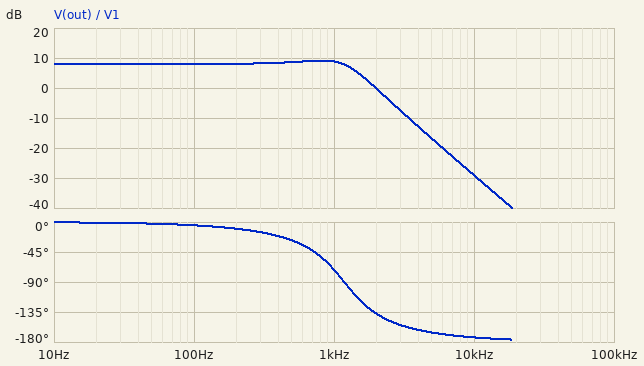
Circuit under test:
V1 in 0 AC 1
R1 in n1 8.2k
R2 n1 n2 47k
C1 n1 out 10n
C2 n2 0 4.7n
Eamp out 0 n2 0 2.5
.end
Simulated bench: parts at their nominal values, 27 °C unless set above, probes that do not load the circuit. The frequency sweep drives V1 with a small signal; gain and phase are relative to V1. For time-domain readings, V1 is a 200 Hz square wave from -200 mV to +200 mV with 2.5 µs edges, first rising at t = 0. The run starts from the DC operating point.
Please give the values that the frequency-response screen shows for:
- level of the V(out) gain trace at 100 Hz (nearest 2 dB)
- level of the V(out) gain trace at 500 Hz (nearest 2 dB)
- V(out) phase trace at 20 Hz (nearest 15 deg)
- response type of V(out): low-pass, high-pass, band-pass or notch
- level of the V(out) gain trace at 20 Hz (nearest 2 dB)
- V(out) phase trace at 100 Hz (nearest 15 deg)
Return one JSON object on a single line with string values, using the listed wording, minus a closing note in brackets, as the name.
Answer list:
{"level of the V(out) gain trace at 100 Hz": "8 dB", "level of the V(out) gain trace at 500 Hz": "8 dB", "V(out) phase trace at 20 Hz": "0 deg", "response type of V(out): low-pass, high-pass, band-pass or notch": "low-pass", "level of the V(out) gain trace at 20 Hz": "8 dB", "V(out) phase trace at 100 Hz": "0 deg"}
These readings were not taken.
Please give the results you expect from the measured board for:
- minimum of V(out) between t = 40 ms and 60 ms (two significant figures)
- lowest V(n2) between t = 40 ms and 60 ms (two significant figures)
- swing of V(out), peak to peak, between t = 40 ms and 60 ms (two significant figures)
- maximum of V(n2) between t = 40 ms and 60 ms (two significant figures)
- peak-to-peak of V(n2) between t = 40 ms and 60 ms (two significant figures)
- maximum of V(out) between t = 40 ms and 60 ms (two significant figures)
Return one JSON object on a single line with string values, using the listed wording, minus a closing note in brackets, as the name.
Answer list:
{"minimum of V(out) between t = 40 ms and 60 ms": "-660 mV", "lowest V(n2) between t = 40 ms and 60 ms": "-260 mV", "swing of V(out), peak to peak, between t = 40 ms and 60 ms": "1.3 V", "maximum of V(n2) between t = 40 ms and 60 ms": "260 mV", "peak-to-peak of V(n2) between t = 40 ms and 60 ms": "530 mV", "maximum of V(out) between t = 40 ms and 60 ms": "660 mV"}
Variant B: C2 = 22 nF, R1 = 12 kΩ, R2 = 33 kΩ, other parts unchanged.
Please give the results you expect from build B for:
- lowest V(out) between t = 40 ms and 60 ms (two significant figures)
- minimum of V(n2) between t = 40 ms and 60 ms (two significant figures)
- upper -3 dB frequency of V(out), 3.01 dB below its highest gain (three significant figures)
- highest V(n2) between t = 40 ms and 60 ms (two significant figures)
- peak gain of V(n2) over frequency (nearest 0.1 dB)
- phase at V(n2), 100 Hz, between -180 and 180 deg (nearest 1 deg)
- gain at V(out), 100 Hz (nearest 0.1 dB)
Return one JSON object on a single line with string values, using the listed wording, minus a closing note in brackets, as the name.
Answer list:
{"lowest V(out) between t = 40 ms and 60 ms": "-470 mV", "minimum of V(n2) between t = 40 ms and 60 ms": "-190 mV", "upper -3 dB frequency of V(out), 3.01 dB below its highest gain": "226 Hz", "highest V(n2) between t = 40 ms and 60 ms": "190 mV", "peak gain of V(n2) over frequency": "0 dB", "phase at V(n2), 100 Hz, between -180 and 180 deg": "-28 deg", "gain at V(out), 100 Hz": "7.2 dB"}
